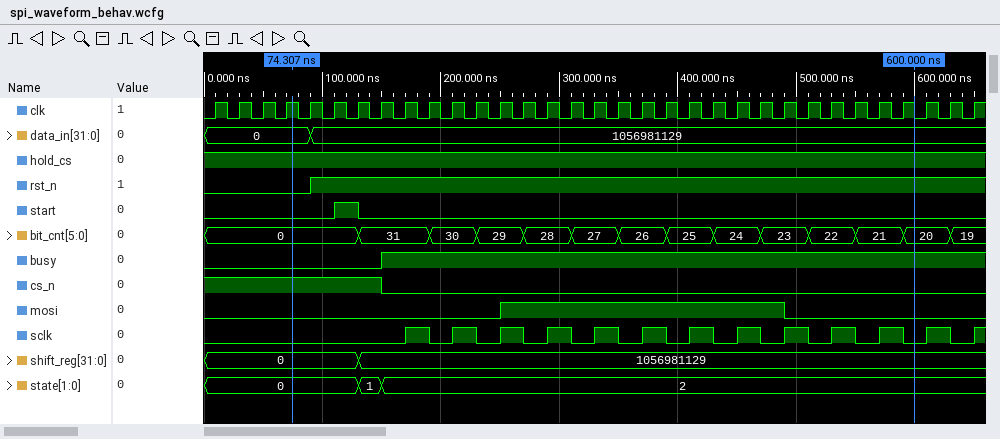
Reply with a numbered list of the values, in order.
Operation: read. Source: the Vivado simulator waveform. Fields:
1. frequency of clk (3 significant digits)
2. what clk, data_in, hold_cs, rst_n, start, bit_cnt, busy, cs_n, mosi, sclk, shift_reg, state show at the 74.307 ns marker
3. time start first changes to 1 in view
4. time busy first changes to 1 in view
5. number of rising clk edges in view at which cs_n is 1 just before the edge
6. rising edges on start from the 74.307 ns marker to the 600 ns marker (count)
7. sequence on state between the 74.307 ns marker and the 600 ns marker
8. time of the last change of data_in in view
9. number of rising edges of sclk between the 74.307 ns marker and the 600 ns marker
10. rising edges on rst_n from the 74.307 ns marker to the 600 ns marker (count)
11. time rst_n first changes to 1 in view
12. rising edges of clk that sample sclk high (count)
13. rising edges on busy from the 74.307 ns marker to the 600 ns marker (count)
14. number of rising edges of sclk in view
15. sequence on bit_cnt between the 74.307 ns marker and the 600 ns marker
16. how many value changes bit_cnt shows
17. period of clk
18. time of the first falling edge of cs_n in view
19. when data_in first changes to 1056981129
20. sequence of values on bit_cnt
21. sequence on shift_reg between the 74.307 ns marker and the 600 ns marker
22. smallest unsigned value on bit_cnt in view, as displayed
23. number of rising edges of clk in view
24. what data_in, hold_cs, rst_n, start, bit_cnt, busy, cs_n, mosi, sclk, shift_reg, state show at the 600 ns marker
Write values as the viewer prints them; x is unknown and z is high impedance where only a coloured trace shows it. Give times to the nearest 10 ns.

1. 50.0 MHz
2. clk=1, data_in=0, hold_cs=1, rst_n=0, start=0, bit_cnt=0, busy=0, cs_n=1, mosi=0, sclk=0, shift_reg=0, state=0
3. 110 ns
4. 150 ns
5. 8
6. 1
7. 0, 1, 2
8. 90 ns
9. 11
10. 1
11. 90 ns
12. 12
13. 1
14. 13
15. 0, 31, 30, 29, 28, 27, 26, 25, 24, 23, 22, 21, 20
16. 13
17. 20 ns
18. 150 ns
19. 90 ns
20. 0, 31, 30, 29, 28, 27, 26, 25, 24, 23, 22, 21, 20, 19
21. 0, 1056981129
22. 0
23. 33
24. data_in=1056981129, hold_cs=1, rst_n=1, start=0, bit_cnt=20, busy=1, cs_n=0, mosi=0, sclk=0, shift_reg=1056981129, state=2
